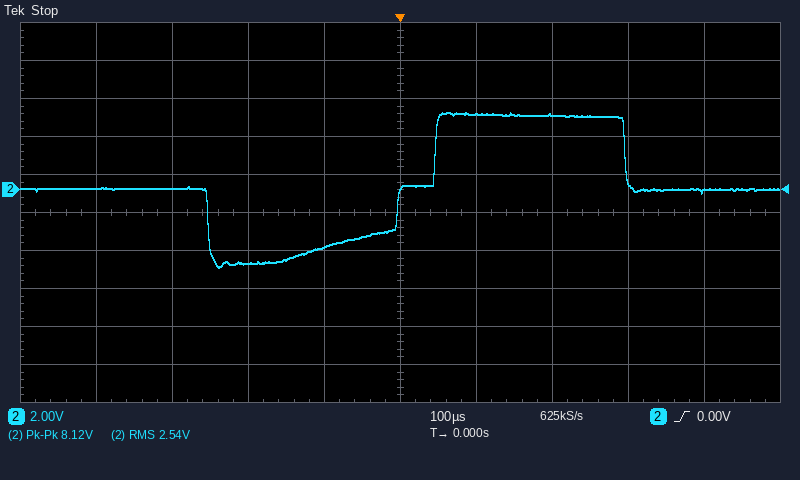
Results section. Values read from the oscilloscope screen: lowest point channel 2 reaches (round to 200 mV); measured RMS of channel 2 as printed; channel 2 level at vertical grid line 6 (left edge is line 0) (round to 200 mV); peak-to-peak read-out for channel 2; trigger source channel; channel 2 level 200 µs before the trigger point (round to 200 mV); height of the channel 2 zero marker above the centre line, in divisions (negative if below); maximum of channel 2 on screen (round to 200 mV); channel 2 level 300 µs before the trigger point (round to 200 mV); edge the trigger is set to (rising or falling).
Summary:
-4.0 V
2.54 V
4.0 V
8.12 V
channel 2
-3.8 V
+0.6 div
4.0 V
0.0 V
rising
